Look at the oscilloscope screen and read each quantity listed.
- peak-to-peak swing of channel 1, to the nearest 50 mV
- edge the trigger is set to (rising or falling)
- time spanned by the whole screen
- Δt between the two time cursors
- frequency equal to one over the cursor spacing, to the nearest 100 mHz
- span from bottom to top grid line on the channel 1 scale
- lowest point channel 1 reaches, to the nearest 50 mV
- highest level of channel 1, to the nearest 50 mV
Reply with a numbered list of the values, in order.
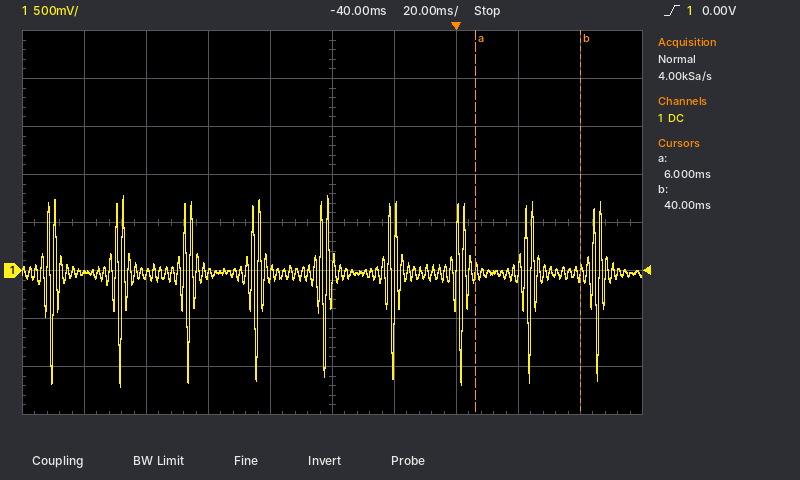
1. 2.00 V
2. rising
3. 200 ms
4. 34 ms
5. 29.4 Hz
6. 4 V
7. -1.20 V
8. 800 mV
